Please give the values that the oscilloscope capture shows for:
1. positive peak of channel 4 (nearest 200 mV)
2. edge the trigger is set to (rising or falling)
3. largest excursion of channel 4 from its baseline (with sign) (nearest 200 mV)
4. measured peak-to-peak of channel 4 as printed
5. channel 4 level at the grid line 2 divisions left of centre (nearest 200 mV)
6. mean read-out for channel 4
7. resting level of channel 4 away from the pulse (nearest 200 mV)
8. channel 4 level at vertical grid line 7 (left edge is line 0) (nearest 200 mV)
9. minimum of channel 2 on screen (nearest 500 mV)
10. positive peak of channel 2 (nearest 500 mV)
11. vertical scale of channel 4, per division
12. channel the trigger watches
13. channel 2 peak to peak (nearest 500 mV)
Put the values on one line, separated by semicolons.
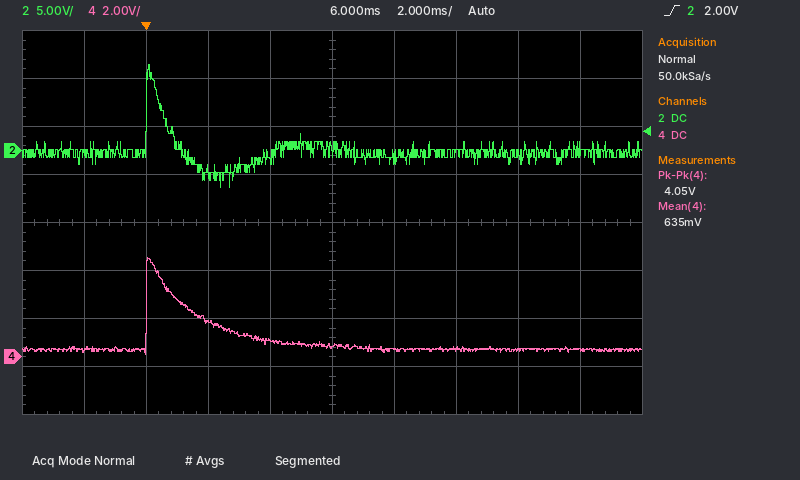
4.2 V; rising; +3.8 V; 4.05 V; 1.4 V; 635 mV; 400 mV; 400 mV; -4.0 V; 9.0 V; 2 V; channel 2; 13.0 V
